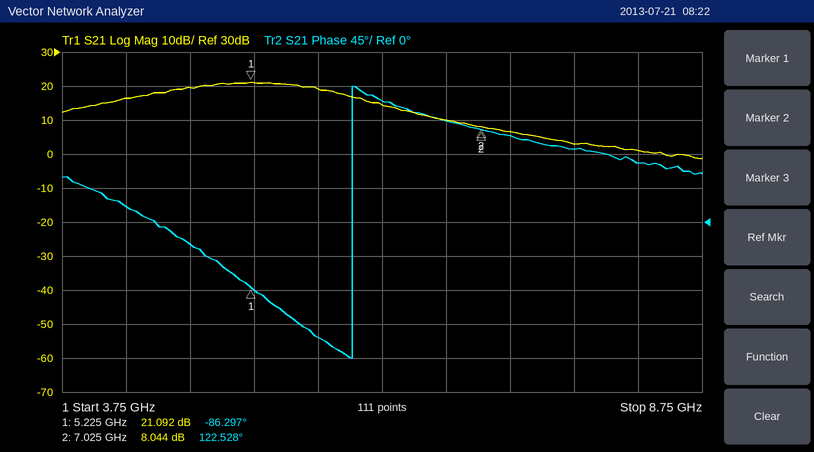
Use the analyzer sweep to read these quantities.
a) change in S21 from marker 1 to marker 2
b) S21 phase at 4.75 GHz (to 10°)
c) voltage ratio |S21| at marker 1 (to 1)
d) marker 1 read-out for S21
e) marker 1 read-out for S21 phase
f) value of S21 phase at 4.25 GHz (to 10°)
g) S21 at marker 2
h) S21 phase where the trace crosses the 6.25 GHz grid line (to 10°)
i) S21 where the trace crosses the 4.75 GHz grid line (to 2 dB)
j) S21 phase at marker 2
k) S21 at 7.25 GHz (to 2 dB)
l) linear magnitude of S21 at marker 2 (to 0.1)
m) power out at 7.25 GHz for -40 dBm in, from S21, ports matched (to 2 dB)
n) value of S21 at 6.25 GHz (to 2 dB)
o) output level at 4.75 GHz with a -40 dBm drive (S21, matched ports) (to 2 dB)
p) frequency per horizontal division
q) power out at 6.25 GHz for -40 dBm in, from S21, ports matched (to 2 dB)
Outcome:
-13.048 dB
-30°
11
21.092 dB
-86.297°
20°
8.044 dB
160°
20 dB
122.528°
6 dB
2.5
-34 dBm
14 dB
-20 dBm
500 MHz
-26 dBm
